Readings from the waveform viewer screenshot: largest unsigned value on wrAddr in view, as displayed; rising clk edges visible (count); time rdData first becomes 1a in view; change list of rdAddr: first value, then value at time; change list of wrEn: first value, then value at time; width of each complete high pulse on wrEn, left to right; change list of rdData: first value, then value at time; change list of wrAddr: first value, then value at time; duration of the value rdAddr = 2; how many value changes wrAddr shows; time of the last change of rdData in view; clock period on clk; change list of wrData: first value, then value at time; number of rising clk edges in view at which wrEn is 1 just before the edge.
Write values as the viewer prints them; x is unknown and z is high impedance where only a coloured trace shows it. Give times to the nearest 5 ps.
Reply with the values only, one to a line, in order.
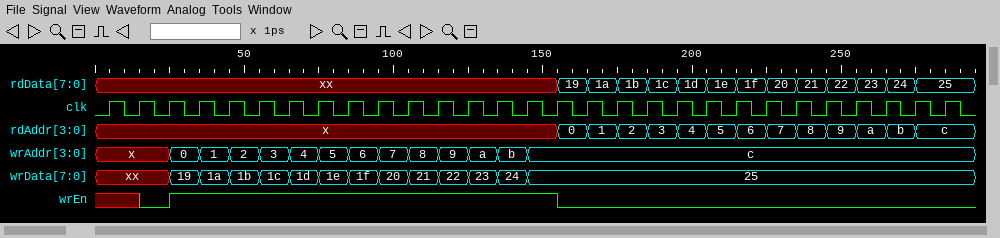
c
29
165 ps
x, 0 at 155 ps, 1 at 165 ps, 2 at 175 ps, 3 at 185 ps, 4 at 195 ps, 5 at 205 ps, 6 at 215 ps, 7 at 225 ps, 8 at 235 ps, 9 at 245 ps, a at 255 ps, b at 265 ps, c at 275 ps
x, 0 at 15 ps, 1 at 25 ps, 0 at 155 ps
130 ps
xx, 19 at 155 ps, 1a at 165 ps, 1b at 175 ps, 1c at 185 ps, 1d at 195 ps, 1e at 205 ps, 1f at 215 ps, 20 at 225 ps, 21 at 235 ps, 22 at 245 ps, 23 at 255 ps, 24 at 265 ps, 25 at 275 ps
x, 0 at 25 ps, 1 at 35 ps, 2 at 45 ps, 3 at 55 ps, 4 at 65 ps, 5 at 75 ps, 6 at 85 ps, 7 at 95 ps, 8 at 105 ps, 9 at 115 ps, a at 125 ps, b at 135 ps, c at 145 ps
10 ps
13
275 ps
10 ps
xx, 19 at 25 ps, 1a at 35 ps, 1b at 45 ps, 1c at 55 ps, 1d at 65 ps, 1e at 75 ps, 1f at 85 ps, 20 at 95 ps, 21 at 105 ps, 22 at 115 ps, 23 at 125 ps, 24 at 135 ps, 25 at 145 ps
13
